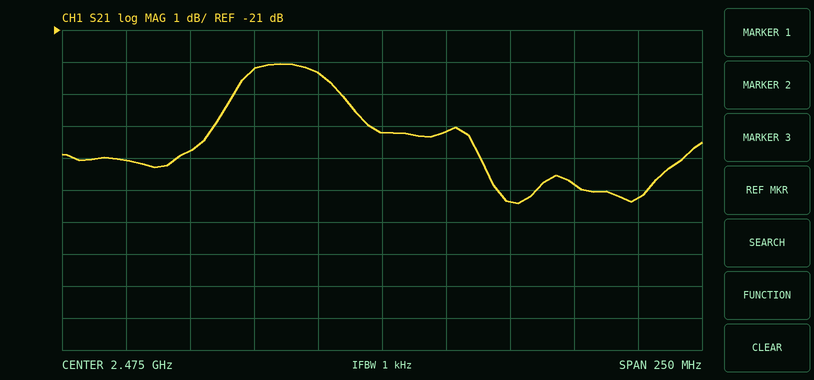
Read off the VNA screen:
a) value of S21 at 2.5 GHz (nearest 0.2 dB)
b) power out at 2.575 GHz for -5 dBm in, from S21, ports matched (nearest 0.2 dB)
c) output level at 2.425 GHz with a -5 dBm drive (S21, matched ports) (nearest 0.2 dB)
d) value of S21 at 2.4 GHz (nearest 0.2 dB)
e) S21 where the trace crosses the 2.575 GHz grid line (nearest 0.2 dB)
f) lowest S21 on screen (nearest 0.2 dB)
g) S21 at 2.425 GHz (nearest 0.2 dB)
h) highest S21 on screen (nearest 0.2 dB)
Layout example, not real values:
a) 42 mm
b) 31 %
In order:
a) -24.2 dB
b) -31.2 dBm
c) -27.2 dBm
d) -24.8 dB
e) -26.2 dB
f) -26.4 dB
g) -22.2 dB
h) -22.0 dB
